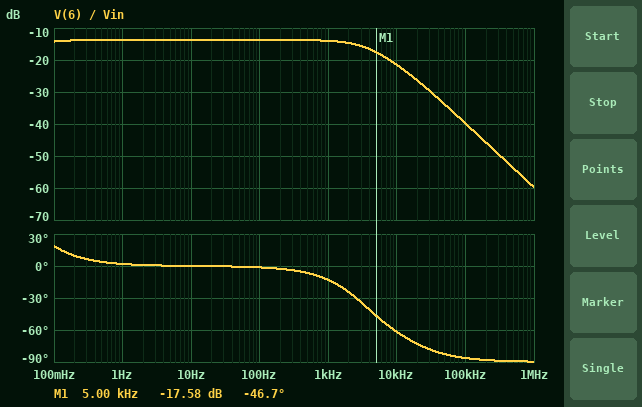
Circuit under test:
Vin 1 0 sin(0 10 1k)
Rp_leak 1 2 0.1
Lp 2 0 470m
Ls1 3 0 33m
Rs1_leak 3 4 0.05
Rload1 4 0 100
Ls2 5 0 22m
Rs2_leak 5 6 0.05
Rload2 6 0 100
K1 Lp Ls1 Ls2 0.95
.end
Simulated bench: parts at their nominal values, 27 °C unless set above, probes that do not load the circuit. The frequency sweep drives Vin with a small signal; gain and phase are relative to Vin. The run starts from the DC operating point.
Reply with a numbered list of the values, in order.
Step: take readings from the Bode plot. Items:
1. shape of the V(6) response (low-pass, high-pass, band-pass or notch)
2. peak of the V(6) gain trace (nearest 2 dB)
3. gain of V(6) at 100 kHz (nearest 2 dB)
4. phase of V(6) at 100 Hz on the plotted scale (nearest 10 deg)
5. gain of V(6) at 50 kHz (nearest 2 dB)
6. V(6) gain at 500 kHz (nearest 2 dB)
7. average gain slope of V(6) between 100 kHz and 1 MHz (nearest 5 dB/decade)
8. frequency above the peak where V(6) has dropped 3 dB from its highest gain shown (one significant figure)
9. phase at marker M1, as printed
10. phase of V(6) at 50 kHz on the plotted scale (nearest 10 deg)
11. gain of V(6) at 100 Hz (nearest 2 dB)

1. low-pass
2. -14 dB
3. -40 dB
4. 0 deg
5. -34 dB
6. -54 dB
7. -20 dB/decade
8. 4 kHz
9. -46.7 deg
10. -80 deg
11. -14 dB
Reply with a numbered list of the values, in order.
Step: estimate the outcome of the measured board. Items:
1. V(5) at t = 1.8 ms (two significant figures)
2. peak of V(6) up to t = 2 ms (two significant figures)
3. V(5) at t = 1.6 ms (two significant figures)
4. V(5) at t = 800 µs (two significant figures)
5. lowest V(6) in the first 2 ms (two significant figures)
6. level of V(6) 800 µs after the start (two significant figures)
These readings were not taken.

1. -2.0 V
2. 2.0 V
3. -780 mV
4. -2.0 V
5. -2.0 V
6. -2.0 V
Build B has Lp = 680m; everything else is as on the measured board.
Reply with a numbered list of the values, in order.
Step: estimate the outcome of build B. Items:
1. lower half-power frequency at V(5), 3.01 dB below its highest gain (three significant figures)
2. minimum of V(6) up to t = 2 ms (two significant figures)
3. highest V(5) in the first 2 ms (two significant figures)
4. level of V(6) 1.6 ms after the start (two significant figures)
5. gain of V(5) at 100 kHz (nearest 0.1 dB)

1. 23.4 mHz
2. -1.7 V
3. 1.7 V
4. -650 mV
5. -41.4 dB
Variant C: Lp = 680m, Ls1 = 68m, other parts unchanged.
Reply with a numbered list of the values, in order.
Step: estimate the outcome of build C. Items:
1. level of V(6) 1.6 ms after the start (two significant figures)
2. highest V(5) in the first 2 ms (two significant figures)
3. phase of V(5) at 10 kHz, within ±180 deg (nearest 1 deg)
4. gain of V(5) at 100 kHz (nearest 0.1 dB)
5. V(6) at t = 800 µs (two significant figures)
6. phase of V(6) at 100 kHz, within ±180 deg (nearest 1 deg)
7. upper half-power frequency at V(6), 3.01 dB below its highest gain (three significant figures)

1. -490 mV
2. 1.6 V
3. -56 deg
4. -41.4 dB
5. -1.6 V
6. -85 deg
7. 2.67 kHz
